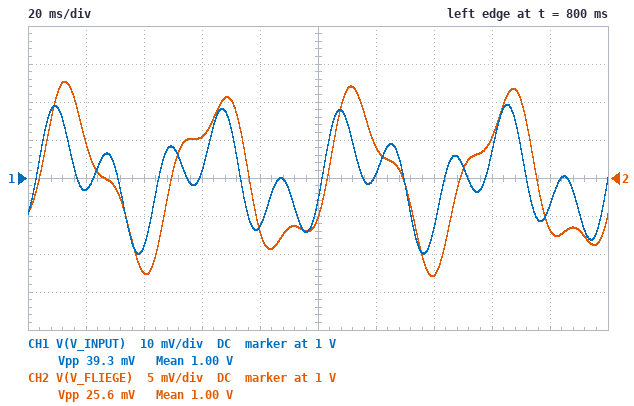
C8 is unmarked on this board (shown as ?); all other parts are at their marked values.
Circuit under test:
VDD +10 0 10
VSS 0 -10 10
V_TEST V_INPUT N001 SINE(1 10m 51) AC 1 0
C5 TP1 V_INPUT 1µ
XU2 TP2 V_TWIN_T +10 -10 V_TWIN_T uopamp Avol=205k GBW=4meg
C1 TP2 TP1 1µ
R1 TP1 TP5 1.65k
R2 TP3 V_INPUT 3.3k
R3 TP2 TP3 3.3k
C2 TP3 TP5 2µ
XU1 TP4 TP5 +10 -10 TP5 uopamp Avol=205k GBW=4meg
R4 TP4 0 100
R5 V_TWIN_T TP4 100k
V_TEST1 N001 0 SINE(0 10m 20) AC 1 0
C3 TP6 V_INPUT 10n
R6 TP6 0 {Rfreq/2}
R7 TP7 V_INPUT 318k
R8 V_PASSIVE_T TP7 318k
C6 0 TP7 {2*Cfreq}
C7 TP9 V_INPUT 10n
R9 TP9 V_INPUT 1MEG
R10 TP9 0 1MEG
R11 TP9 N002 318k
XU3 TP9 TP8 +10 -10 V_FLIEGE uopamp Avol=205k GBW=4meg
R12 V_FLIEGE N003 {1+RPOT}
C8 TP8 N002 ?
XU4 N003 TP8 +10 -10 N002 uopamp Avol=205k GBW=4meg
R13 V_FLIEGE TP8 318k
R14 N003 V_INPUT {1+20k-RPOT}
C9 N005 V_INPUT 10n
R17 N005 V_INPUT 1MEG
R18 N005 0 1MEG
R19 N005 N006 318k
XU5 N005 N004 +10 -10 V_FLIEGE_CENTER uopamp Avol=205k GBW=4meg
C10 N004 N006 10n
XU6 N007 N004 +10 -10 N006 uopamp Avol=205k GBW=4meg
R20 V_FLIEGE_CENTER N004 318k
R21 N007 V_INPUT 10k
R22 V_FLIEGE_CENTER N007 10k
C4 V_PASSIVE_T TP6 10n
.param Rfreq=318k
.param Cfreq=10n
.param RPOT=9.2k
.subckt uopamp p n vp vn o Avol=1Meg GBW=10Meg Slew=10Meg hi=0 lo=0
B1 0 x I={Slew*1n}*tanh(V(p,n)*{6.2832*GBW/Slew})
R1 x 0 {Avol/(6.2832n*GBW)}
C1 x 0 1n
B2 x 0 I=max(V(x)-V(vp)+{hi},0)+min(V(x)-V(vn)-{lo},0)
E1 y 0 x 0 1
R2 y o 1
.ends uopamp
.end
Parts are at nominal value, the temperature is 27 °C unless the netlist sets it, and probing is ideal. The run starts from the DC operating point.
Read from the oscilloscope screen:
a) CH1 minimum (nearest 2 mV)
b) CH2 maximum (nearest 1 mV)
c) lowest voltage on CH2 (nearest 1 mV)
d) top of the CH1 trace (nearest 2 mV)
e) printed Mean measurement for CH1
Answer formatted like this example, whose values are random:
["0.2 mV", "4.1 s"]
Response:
["980 mV", "1.013 V", "987 mV", "1.020 V", "1.00 V"]
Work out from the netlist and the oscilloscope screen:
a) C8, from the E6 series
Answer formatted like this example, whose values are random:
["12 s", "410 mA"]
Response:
["6.8 nF"]
